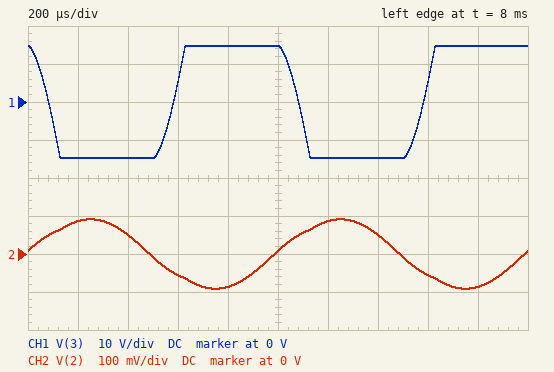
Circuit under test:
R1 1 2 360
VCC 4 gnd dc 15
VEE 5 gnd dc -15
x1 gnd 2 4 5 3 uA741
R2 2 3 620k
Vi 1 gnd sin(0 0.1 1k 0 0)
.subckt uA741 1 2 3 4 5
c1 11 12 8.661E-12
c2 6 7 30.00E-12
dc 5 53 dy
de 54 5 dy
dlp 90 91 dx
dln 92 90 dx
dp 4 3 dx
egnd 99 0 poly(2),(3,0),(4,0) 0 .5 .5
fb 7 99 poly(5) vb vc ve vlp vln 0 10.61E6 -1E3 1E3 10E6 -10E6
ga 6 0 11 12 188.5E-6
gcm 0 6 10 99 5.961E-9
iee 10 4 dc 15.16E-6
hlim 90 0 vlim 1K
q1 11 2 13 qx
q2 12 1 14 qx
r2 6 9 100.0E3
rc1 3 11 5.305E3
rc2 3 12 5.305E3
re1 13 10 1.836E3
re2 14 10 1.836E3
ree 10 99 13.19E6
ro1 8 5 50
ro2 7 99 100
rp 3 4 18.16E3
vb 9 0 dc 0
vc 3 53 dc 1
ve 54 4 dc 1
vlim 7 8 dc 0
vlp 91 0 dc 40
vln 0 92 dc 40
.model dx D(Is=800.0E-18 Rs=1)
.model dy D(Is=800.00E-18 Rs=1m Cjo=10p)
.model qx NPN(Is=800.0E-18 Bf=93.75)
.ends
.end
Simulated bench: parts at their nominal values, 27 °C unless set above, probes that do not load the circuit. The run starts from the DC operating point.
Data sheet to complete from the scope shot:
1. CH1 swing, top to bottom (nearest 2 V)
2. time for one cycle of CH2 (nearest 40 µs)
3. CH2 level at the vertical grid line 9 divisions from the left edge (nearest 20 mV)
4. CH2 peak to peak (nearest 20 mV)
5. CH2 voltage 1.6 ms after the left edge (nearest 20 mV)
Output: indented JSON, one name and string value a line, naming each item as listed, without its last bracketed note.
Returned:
{
  "CH1 swing, top to bottom": "30 V",
  "time for one cycle of CH2": "1.00 ms",
  "CH2 level at the vertical grid line 9 divisions from the left edge": "-80 mV",
  "CH2 peak to peak": "180 mV",
  "CH2 voltage 1.6 ms after the left edge": "-60 mV"
}
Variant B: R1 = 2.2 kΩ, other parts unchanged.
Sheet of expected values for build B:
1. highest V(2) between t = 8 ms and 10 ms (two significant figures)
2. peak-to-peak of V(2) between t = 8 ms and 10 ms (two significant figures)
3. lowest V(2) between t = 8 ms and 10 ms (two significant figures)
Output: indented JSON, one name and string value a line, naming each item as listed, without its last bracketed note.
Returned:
{
  "highest V(2) between t = 8 ms and 10 ms": "47 mV",
  "peak-to-peak of V(2) between t = 8 ms and 10 ms": "94 mV",
  "lowest V(2) between t = 8 ms and 10 ms": "-47 mV"
}
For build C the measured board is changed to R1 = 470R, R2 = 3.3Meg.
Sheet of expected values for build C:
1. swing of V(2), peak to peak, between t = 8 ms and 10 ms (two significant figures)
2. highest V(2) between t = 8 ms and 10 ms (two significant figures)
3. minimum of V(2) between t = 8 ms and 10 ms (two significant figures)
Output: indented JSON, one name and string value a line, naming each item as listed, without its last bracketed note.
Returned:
{
  "swing of V(2), peak to peak, between t = 8 ms and 10 ms": "200 mV",
  "highest V(2) between t = 8 ms and 10 ms": "98 mV",
  "minimum of V(2) between t = 8 ms and 10 ms": "-98 mV"
}
